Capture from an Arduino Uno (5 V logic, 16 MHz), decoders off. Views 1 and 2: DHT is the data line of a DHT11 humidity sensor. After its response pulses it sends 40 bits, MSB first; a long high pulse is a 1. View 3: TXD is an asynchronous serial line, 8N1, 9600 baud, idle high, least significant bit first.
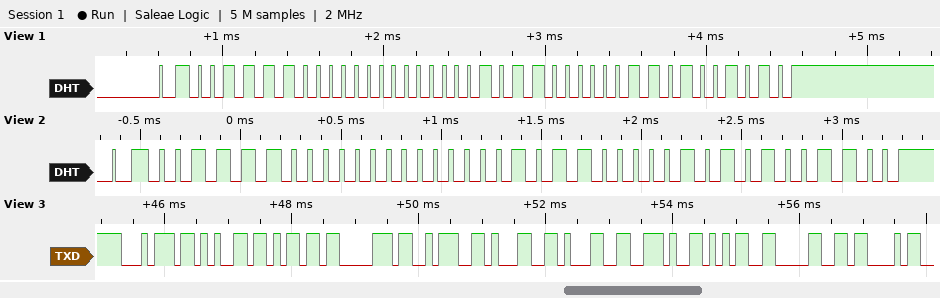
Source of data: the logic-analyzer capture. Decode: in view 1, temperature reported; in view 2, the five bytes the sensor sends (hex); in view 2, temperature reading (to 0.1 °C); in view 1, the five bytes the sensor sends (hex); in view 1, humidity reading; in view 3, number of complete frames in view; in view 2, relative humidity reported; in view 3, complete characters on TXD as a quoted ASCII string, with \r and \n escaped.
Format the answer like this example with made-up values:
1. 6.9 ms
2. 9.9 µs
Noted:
1. 11.3 °C
2. 3C 00 0B 05 4C
3. 11.5 °C
4. 3C 00 0B 03 4A
5. 60 %
6. 11
7. 60 %
8. "temp:11.50C"
